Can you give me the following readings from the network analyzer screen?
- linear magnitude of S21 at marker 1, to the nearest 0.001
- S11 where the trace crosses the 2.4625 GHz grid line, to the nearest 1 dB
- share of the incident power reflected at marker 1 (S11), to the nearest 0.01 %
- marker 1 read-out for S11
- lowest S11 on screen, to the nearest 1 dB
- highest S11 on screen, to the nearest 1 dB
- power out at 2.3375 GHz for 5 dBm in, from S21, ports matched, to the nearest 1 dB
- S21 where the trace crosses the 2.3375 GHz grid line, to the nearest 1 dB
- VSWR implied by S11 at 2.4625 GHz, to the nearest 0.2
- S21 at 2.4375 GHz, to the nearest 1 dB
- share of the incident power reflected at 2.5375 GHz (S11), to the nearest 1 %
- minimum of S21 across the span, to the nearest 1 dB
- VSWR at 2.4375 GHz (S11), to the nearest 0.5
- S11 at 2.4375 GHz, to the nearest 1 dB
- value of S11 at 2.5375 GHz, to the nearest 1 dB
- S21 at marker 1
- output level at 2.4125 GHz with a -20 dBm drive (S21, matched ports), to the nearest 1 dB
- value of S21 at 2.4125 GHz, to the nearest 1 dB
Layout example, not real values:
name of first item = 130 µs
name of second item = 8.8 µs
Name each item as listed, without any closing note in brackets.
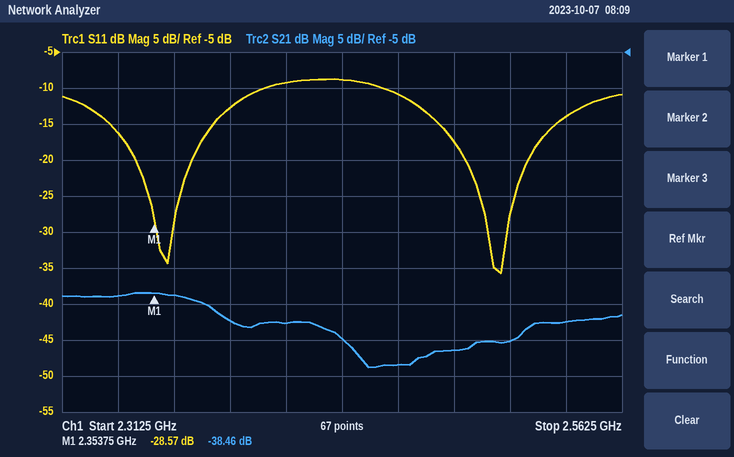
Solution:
linear magnitude of S21 at marker 1, to the nearest 0.001 = 0.012
S11 where the trace crosses the 2.4625 GHz grid line, to the nearest 1 dB = -11 dB
share of the incident power reflected at marker 1 (S11), to the nearest 0.01 % = 0.14 %
marker 1 read-out for S11 = -28.57 dB
lowest S11 on screen, to the nearest 1 dB = -36 dB
highest S11 on screen, to the nearest 1 dB = -9 dB
power out at 2.3375 GHz for 5 dBm in, from S21, ports matched, to the nearest 1 dB = -34 dBm
S21 where the trace crosses the 2.3375 GHz grid line, to the nearest 1 dB = -39 dB
VSWR implied by S11 at 2.4625 GHz, to the nearest 0.2 = 1.8
S21 at 2.4375 GHz, to the nearest 1 dB = -45 dB
share of the incident power reflected at 2.5375 GHz (S11), to the nearest 1 % = 4 %
minimum of S21 across the span, to the nearest 1 dB = -49 dB
VSWR at 2.4375 GHz (S11), to the nearest 0.5 = 2.0
S11 at 2.4375 GHz, to the nearest 1 dB = -9 dB
value of S11 at 2.5375 GHz, to the nearest 1 dB = -14 dB
S21 at marker 1 = -38.46 dB
output level at 2.4125 GHz with a -20 dBm drive (S21, matched ports), to the nearest 1 dB = -63 dBm
value of S21 at 2.4125 GHz, to the nearest 1 dB = -43 dB
